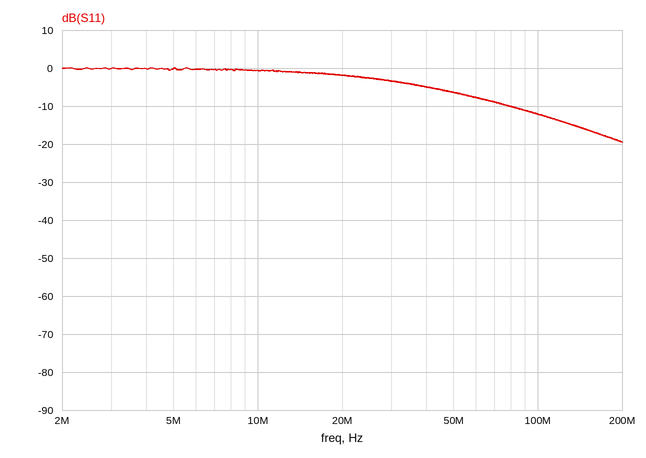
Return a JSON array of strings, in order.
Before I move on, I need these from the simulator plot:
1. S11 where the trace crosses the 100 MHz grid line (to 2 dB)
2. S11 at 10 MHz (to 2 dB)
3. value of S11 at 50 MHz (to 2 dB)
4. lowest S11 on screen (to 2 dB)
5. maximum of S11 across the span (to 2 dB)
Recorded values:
["-12 dB", "0 dB", "-6 dB", "-20 dB", "0 dB"]
